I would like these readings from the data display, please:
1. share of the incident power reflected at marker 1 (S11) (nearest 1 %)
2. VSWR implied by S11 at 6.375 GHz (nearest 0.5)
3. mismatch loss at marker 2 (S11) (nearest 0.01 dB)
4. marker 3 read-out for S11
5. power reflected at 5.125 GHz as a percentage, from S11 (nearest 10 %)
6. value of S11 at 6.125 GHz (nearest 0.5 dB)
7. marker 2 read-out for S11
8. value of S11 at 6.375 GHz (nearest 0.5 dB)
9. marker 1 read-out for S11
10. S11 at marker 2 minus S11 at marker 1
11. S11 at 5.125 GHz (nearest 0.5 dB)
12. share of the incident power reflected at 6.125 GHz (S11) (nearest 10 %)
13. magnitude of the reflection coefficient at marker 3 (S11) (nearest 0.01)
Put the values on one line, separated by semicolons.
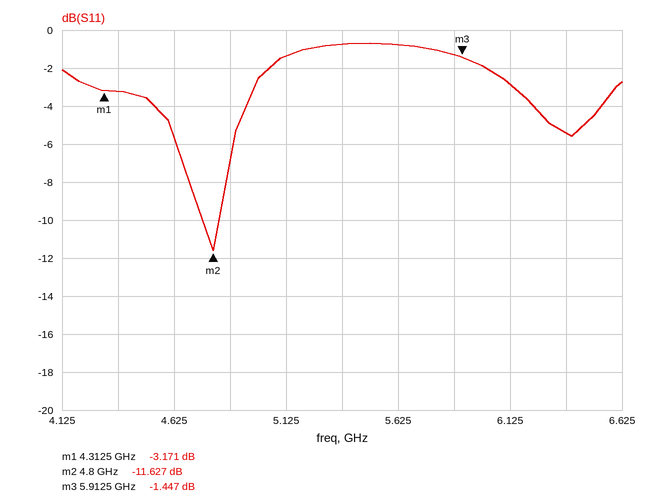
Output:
48 %; 3.5; 0.31 dB; -1.447 dB; 70 %; -3.0 dB; -11.627 dB; -5.5 dB; -3.171 dB; -8.456 dB; -1.5 dB; 50 %; 0.85
